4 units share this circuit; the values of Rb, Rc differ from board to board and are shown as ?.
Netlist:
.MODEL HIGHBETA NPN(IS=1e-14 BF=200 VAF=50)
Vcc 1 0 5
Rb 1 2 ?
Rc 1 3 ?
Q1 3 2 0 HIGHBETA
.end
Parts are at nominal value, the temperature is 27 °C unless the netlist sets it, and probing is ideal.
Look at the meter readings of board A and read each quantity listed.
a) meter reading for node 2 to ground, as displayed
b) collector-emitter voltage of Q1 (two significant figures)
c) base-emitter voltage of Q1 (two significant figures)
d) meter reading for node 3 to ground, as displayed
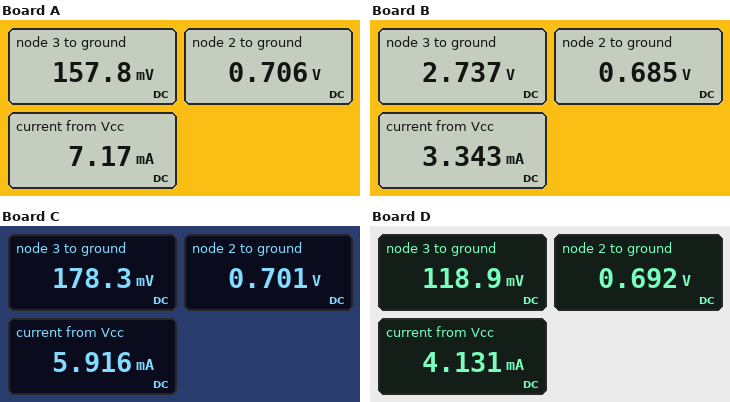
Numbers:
0.706 V
160 mV
710 mV
157.8 mV
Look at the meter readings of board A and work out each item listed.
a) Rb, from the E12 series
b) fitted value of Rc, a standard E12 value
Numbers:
82 kΩ
680 Ω
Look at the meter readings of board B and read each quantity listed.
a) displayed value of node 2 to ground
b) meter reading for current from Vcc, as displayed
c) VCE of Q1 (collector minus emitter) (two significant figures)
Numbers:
0.685 V
3.343 mA
2.7 V
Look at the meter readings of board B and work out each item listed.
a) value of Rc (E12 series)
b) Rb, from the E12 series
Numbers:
680 Ω
270 kΩ
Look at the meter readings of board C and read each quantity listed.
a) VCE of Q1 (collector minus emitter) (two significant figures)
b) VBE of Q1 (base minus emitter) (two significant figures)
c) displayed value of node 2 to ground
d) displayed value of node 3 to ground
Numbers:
180 mV
700 mV
0.701 V
178.3 mV
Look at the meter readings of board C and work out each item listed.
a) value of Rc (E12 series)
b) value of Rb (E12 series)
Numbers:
820 Ω
120 kΩ
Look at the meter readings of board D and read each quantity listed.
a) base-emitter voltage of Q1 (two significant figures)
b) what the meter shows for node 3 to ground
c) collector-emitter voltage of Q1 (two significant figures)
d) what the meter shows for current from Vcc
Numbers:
690 mV
118.9 mV
120 mV
4.131 mA
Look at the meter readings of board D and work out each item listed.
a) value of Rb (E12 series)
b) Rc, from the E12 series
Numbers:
68 kΩ
1.2 kΩ
